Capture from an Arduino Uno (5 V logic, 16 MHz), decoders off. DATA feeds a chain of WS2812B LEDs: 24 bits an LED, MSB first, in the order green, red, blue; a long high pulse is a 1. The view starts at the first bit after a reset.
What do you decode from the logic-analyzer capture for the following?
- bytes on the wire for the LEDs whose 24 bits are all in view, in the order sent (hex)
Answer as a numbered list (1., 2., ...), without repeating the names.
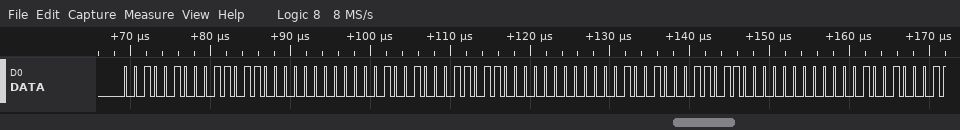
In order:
1. 24 6C 00 24 6C 00 24 6C 00
